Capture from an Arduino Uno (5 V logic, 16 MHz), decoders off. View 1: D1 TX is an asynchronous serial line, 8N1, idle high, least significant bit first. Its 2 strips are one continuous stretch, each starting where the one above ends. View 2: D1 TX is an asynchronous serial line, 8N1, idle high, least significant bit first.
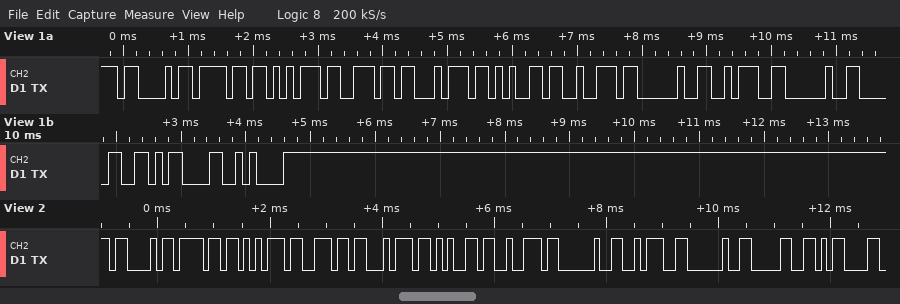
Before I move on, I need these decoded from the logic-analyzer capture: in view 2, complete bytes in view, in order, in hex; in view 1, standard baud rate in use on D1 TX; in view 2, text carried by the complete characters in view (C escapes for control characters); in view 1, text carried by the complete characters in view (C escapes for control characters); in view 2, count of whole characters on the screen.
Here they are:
43 6F 75 6E 74 65 72 20 3A 20 30 0D
9600 baud
"Counter : 0\r"
"Counter : 0\r\n"
12
